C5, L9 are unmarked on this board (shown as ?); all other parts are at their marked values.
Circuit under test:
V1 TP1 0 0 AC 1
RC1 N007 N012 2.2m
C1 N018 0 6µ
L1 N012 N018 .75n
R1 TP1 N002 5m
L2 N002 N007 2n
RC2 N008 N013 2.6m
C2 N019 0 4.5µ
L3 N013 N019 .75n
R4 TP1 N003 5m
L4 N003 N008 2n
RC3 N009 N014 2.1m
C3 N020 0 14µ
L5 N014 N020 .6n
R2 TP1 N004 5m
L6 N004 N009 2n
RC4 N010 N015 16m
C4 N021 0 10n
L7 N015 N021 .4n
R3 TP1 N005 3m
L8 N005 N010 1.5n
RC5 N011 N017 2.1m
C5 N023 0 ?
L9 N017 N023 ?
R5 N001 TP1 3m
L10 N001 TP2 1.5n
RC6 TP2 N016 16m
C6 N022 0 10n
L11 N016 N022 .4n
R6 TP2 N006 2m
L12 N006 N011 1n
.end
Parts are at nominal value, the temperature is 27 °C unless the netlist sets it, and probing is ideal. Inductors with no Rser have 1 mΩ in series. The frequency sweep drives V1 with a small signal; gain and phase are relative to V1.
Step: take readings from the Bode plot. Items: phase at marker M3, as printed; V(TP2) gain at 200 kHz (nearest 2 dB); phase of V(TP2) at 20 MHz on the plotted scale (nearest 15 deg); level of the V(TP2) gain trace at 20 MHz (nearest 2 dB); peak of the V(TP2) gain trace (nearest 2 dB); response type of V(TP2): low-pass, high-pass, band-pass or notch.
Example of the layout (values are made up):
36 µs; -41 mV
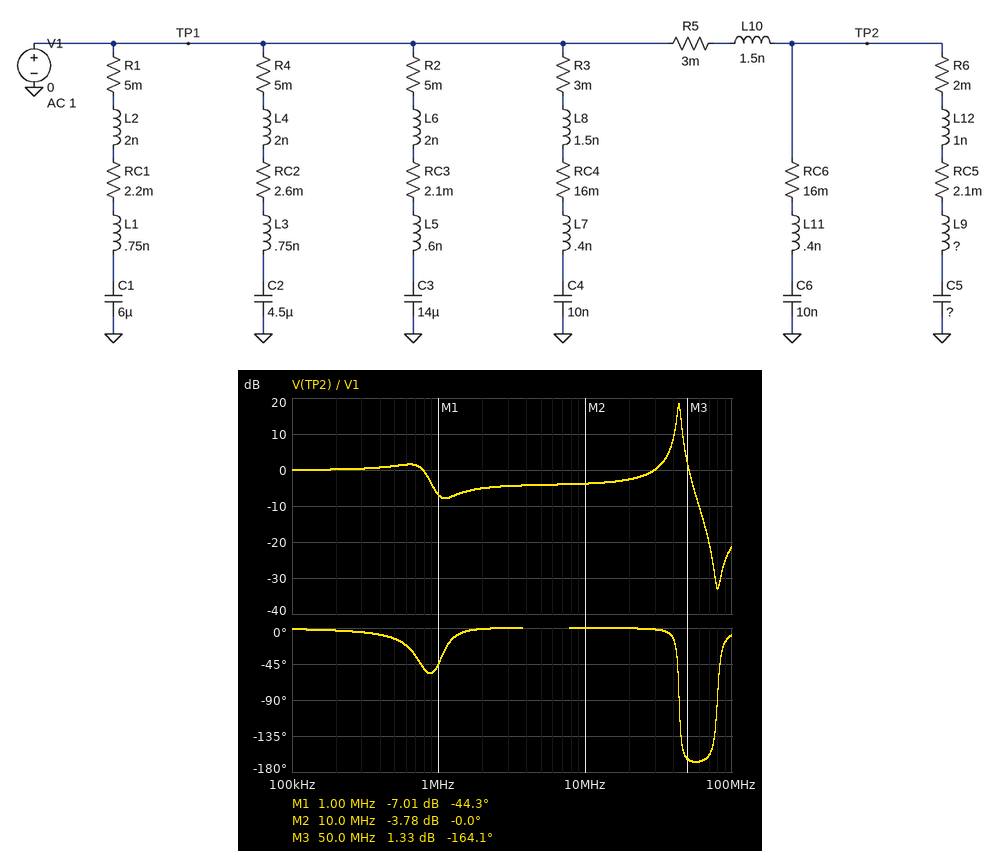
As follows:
-164.1 deg; 0 dB; 0 deg; -2 dB; 18 dB; band-pass
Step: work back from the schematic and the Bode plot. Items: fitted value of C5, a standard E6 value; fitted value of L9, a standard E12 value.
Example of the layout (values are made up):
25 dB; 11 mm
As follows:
10 µF; 1.5 nH
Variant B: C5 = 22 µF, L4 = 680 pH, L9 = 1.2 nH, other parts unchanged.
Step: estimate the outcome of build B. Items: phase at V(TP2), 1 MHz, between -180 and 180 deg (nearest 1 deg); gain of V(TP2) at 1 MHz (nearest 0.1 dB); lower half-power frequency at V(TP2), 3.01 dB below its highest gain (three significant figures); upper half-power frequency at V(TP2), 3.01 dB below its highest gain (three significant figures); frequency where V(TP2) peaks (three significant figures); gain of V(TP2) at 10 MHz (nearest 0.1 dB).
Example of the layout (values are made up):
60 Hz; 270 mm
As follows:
-11 deg; -6.5 dB; 43.0 MHz; 45.4 MHz; 44.2 MHz; -4.2 dB
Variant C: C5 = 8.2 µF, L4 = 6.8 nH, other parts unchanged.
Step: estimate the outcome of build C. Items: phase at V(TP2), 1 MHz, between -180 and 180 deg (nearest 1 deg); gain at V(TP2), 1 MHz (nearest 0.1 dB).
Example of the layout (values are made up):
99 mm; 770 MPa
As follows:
-61 deg; -4.2 dB
